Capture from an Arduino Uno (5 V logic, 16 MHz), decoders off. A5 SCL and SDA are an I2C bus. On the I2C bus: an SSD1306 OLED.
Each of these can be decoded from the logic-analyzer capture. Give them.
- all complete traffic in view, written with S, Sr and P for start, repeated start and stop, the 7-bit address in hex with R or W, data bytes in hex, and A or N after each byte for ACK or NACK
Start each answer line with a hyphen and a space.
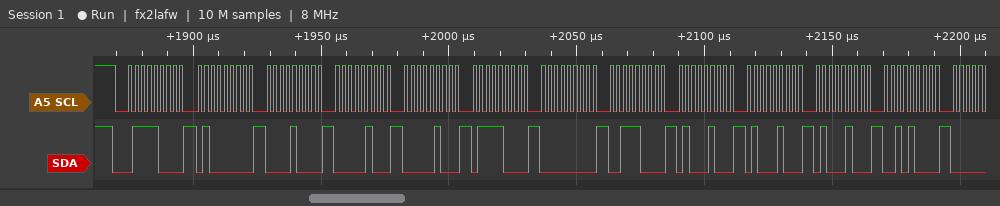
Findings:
- S 3CW A 40 A 08 A 04 A 04 A 78 A 00 A 38 A 44 A 44 A 44 A 28 A
